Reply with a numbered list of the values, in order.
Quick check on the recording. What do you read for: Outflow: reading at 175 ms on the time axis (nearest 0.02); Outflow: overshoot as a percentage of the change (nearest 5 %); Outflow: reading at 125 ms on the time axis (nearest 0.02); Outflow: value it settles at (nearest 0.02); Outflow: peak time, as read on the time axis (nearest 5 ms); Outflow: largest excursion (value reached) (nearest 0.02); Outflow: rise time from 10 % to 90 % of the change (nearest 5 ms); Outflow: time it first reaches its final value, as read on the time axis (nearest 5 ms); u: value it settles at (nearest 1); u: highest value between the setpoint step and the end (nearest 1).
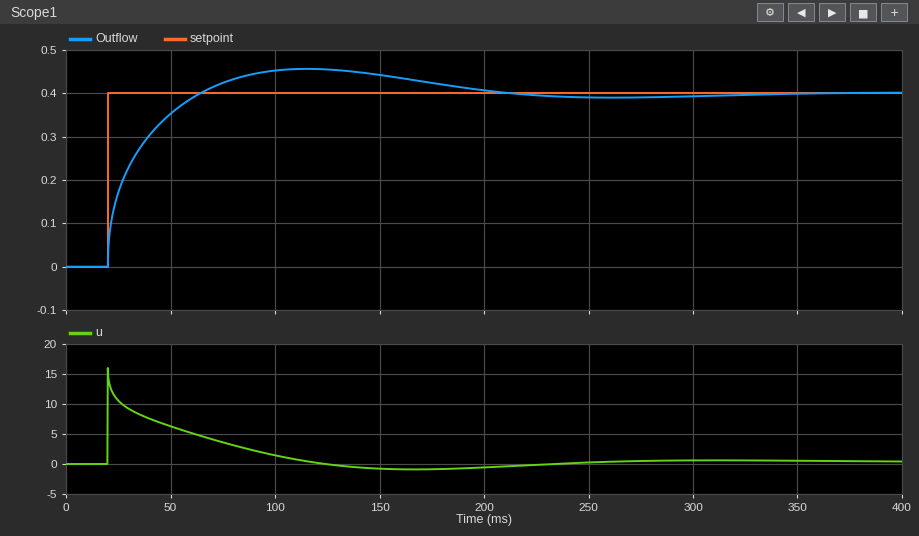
1. 0.42
2. 15 %
3. 0.46
4. 0.40
5. 115 ms
6. 0.46
7. 30 ms
8. 65 ms
9. 0
10. 16
